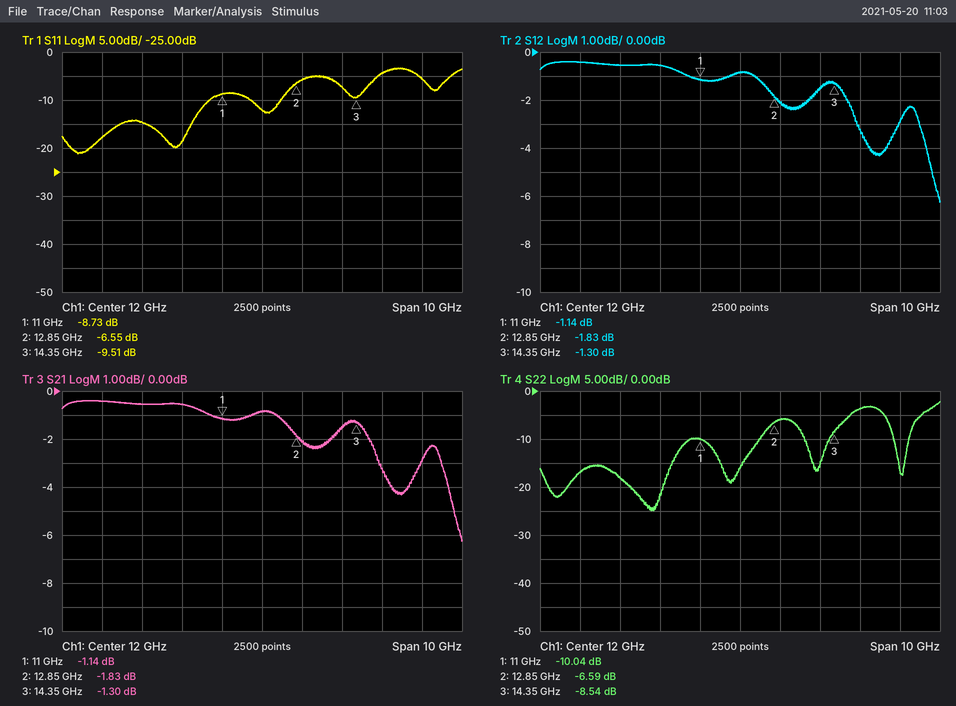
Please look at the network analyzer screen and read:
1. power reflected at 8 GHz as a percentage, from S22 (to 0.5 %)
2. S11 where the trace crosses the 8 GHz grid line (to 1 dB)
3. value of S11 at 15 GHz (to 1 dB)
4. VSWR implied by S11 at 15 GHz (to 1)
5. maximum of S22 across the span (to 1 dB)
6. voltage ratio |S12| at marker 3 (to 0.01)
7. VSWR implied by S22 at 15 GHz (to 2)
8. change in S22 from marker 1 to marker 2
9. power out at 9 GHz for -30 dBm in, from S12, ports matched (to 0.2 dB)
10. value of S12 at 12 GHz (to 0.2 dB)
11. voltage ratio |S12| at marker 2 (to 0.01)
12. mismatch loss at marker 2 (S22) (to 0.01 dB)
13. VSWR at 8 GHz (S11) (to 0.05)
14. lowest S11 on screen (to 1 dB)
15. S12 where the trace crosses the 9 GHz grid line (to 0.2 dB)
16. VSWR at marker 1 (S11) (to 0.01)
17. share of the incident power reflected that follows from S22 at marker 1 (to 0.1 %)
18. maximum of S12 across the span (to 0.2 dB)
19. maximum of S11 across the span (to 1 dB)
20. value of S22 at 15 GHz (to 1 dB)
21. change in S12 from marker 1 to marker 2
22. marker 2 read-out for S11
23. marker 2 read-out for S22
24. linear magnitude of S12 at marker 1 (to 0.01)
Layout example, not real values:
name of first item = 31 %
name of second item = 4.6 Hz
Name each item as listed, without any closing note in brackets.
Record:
power reflected at 8 GHz as a percentage, from S22 = 2.0 %
S11 where the trace crosses the 8 GHz grid line = -18 dB
value of S11 at 15 GHz = -4 dB
VSWR implied by S11 at 15 GHz = 4
maximum of S22 across the span = -2 dB
voltage ratio |S12| at marker 3 = 0.86
VSWR implied by S22 at 15 GHz = 4
change in S22 from marker 1 to marker 2 = 3.45 dB
power out at 9 GHz for -30 dBm in, from S12, ports matched = -30.6 dBm
value of S12 at 12 GHz = -0.8 dB
voltage ratio |S12| at marker 2 = 0.81
mismatch loss at marker 2 (S22) = 1.08 dB
VSWR at 8 GHz (S11) = 1.30
lowest S11 on screen = -21 dB
S12 where the trace crosses the 9 GHz grid line = -0.6 dB
VSWR at marker 1 (S11) = 2.15
share of the incident power reflected that follows from S22 at marker 1 = 9.9 %
maximum of S12 across the span = -0.4 dB
maximum of S11 across the span = -3 dB
value of S22 at 15 GHz = -4 dB
change in S12 from marker 1 to marker 2 = -0.69 dB
marker 2 read-out for S11 = -6.55 dB
marker 2 read-out for S22 = -6.59 dB
linear magnitude of S12 at marker 1 = 0.88
